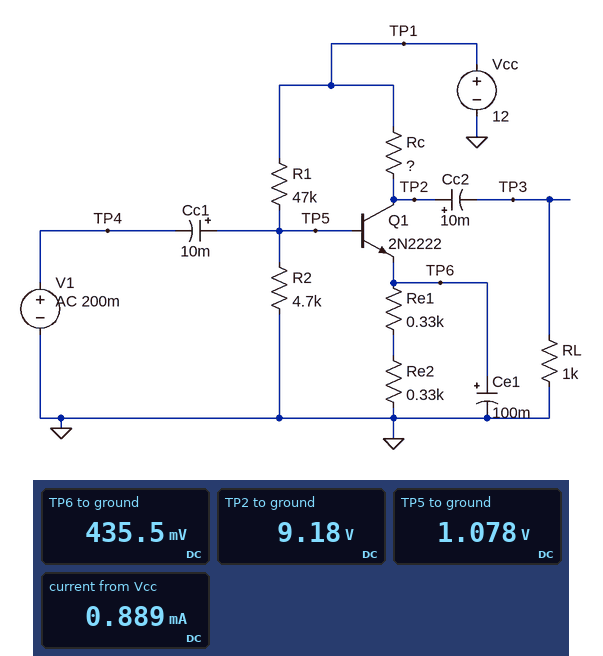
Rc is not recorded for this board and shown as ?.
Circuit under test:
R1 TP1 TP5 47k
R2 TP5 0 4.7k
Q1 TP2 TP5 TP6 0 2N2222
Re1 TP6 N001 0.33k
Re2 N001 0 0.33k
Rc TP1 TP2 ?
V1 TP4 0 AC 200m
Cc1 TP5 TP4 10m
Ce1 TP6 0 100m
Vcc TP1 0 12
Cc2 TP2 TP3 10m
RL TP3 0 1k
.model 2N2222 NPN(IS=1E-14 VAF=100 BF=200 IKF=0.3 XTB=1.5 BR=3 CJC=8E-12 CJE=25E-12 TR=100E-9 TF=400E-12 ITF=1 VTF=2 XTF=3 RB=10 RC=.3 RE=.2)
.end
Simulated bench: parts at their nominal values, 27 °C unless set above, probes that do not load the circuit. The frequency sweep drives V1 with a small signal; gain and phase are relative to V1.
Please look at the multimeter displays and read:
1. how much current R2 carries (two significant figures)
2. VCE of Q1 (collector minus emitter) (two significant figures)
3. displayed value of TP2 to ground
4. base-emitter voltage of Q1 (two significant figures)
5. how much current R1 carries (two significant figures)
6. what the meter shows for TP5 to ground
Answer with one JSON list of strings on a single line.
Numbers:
["230 µA", "8.7 V", "9.18 V", "640 mV", "230 µA", "1.078 V"]
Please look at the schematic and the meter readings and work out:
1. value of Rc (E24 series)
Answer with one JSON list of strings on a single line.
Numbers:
["4.3 kΩ"]
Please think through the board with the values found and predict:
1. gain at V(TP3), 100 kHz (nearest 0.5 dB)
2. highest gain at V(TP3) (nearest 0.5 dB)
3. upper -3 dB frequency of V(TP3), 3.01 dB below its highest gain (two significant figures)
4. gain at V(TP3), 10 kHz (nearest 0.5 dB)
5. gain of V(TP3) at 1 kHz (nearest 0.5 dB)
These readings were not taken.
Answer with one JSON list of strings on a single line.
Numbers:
["26.0 dB", "26.0 dB", "42 MHz", "26.0 dB", "26.0 dB"]
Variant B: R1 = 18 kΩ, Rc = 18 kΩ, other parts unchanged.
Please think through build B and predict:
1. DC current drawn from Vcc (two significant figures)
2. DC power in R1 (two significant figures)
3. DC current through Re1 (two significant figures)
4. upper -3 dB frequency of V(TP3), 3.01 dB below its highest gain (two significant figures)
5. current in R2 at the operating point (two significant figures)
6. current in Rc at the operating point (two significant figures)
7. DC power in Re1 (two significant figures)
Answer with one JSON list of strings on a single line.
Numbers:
["1.2 mA", "6.4 mW", "950 µA", "400 MHz", "280 µA", "630 µA", "300 µW"]
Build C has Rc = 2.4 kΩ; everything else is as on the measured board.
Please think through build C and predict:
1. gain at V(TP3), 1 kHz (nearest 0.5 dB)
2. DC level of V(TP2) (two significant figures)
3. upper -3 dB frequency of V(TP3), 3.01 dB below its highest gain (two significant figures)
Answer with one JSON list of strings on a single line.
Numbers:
["25.0 dB", "10 V", "50 MHz"]
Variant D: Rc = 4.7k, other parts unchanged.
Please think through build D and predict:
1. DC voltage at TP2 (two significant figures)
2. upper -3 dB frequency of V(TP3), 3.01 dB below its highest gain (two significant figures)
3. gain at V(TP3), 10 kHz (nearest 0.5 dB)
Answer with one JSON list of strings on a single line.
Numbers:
["8.9 V", "41 MHz", "26.5 dB"]
